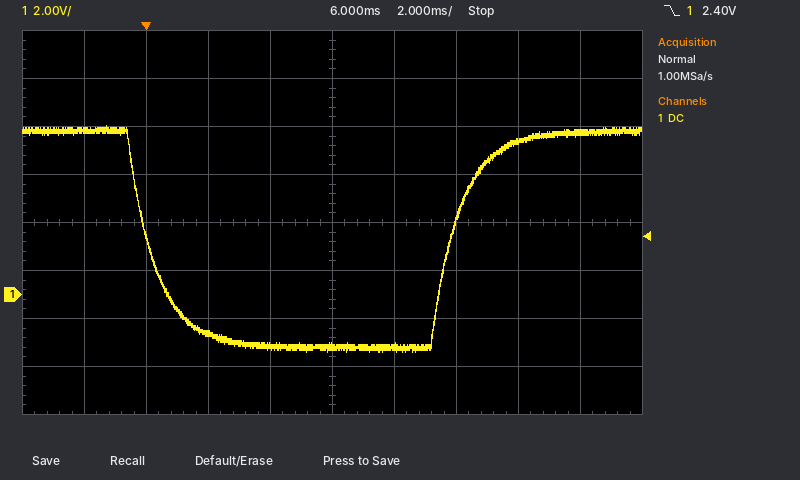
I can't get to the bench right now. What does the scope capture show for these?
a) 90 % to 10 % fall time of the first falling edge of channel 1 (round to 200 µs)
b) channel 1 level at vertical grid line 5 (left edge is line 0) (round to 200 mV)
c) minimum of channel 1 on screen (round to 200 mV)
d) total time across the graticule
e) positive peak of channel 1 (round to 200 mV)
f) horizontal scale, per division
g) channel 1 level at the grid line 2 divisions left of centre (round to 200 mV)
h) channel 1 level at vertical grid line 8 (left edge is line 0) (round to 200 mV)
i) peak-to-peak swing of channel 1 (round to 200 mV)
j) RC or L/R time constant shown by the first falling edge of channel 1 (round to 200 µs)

2.0 ms
-2.2 V
-2.4 V
20 ms
7.0 V
2 ms
-1.6 V
6.4 V
9.4 V
1.0 ms
